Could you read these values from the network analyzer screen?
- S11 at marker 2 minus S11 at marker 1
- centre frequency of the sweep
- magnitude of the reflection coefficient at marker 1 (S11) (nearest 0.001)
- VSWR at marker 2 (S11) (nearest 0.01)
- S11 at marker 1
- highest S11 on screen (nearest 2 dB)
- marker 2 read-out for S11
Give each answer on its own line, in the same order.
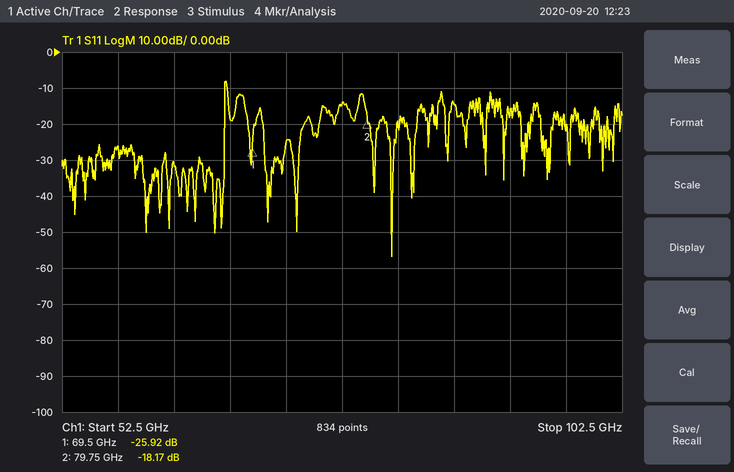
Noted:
7.75 dB
77.5 GHz
0.051
1.28
-25.92 dB
-8 dB
-18.17 dB
